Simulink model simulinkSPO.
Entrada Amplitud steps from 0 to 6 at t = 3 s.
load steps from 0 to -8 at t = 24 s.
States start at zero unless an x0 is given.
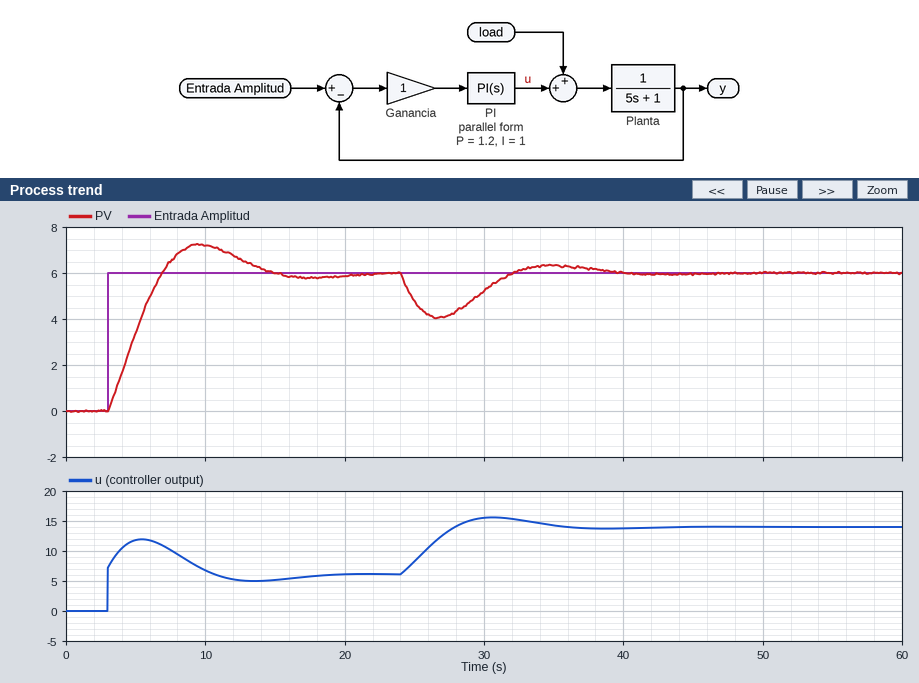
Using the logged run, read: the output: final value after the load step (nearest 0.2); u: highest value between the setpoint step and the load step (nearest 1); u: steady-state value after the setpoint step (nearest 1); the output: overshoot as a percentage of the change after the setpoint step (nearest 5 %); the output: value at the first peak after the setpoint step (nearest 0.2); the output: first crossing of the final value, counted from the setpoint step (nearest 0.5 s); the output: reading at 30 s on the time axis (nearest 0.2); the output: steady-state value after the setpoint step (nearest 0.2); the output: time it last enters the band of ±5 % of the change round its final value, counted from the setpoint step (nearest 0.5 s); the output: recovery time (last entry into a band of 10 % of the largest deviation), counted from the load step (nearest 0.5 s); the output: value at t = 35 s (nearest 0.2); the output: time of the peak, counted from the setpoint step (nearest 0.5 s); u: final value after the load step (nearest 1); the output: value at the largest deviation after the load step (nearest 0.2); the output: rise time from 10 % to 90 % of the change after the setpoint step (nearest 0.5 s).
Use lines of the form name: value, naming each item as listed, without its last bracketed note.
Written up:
the output: final value after the load step: 6.0
u: highest value between the setpoint step and the load step: 12
u: steady-state value after the setpoint step: 6
the output: overshoot as a percentage of the change after the setpoint step: 20 %
the output: value at the first peak after the setpoint step: 7.2
the output: first crossing of the final value, counted from the setpoint step: 4.0 s
the output: reading at 30 s on the time axis: 5.2
the output: steady-state value after the setpoint step: 6.0
the output: time it last enters the band of ±5 % of the change round its final value, counted from the setpoint step: 10.5 s
the output: recovery time (last entry into a band of 10 % of the largest deviation), counted from the load step: 13.5 s
the output: value at t = 35 s: 6.4
the output: time of the peak, counted from the setpoint step: 6.5 s
u: final value after the load step: 14
the output: value at the largest deviation after the load step: 4.0
the output: rise time from 10 % to 90 % of the change after the setpoint step: 3.0 s
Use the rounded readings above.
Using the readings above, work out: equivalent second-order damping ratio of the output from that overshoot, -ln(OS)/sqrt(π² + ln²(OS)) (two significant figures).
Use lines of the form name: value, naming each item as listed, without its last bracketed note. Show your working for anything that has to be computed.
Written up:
equivalent second-order damping ratio of the output from that overshoot, -ln(OS)/sqrt(π² + ln²(OS)): ln(0.2) = -1.609; 1.609 / sqrt(9.870 + 2.590) = 0.46
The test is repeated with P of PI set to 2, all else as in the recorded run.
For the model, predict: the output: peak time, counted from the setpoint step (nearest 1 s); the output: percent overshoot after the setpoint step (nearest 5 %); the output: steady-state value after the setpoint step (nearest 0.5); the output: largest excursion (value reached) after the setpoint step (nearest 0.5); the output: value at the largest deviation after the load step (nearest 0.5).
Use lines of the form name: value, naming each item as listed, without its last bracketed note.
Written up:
the output: peak time, counted from the setpoint step: 6 s
the output: percent overshoot after the setpoint step: 10 %
the output: steady-state value after the setpoint step: 6.0
the output: largest excursion (value reached) after the setpoint step: 6.5
the output: value at the largest deviation after the load step: 4.5
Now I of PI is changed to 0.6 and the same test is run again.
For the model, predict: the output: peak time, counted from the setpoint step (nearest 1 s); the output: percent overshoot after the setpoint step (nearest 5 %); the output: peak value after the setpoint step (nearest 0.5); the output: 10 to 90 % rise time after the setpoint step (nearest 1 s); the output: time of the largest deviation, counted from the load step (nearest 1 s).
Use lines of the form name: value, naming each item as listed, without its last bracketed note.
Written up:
the output: peak time, counted from the setpoint step: 9 s
the output: percent overshoot after the setpoint step: 10 %
the output: peak value after the setpoint step: 6.5
the output: 10 to 90 % rise time after the setpoint step: 4 s
the output: time of the largest deviation, counted from the load step: 3 s
